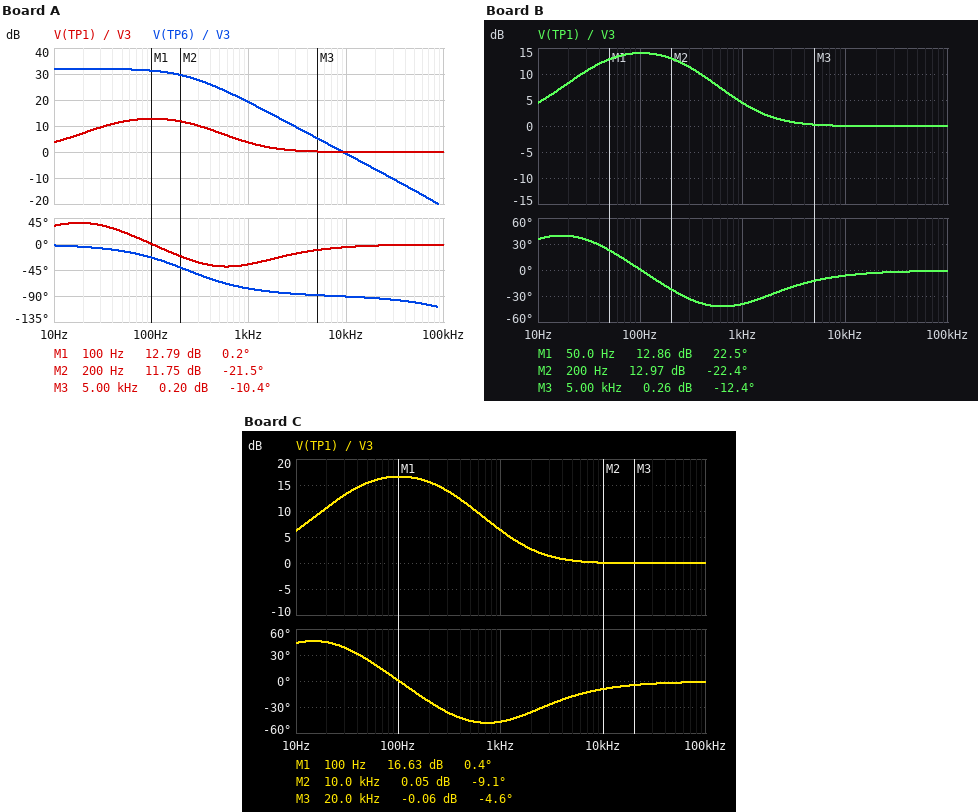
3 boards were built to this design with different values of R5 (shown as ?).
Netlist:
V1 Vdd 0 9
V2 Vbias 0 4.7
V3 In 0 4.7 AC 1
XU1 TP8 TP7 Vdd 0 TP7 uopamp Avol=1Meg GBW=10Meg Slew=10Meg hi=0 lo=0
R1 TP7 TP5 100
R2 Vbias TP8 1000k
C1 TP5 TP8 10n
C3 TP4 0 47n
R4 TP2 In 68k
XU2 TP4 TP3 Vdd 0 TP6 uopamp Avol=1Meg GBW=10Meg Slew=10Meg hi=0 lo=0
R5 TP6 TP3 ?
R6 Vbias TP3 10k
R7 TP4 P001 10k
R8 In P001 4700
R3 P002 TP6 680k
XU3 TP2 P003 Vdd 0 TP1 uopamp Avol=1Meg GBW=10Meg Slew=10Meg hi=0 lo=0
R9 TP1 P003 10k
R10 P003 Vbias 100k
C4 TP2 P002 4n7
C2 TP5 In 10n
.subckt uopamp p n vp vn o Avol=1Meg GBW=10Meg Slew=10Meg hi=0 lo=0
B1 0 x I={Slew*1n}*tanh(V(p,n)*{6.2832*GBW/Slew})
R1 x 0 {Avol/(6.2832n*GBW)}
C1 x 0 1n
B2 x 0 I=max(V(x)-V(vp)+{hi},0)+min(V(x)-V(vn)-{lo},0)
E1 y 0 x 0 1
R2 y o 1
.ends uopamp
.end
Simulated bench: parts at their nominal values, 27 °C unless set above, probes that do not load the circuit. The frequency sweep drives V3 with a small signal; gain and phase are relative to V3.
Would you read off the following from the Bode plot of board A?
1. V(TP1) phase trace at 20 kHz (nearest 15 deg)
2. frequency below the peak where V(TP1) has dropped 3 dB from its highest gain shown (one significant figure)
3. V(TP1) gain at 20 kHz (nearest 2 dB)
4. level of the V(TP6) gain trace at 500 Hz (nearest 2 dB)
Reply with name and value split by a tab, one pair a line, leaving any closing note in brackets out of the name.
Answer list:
V(TP1) phase trace at 20 kHz	0 deg
frequency below the peak where V(TP1) has dropped 3 dB from its highest gain shown	30 Hz
V(TP1) gain at 20 kHz	0 dB
level of the V(TP6) gain trace at 500 Hz	24 dB
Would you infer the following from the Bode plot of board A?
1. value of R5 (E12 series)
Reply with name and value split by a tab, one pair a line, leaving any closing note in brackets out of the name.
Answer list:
value of R5	390 kΩ
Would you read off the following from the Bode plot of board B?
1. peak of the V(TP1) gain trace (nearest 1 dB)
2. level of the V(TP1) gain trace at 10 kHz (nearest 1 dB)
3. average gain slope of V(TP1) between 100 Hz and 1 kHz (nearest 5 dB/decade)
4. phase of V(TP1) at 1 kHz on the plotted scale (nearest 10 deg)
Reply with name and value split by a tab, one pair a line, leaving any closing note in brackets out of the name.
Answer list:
peak of the V(TP1) gain trace	14 dB
level of the V(TP1) gain trace at 10 kHz	0 dB
average gain slope of V(TP1) between 100 Hz and 1 kHz	-10 dB/decade
phase of V(TP1) at 1 kHz on the plotted scale	-40 deg
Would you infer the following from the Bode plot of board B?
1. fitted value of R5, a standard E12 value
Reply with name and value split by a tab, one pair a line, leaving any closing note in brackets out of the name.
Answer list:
fitted value of R5, a standard E12 value	470 kΩ
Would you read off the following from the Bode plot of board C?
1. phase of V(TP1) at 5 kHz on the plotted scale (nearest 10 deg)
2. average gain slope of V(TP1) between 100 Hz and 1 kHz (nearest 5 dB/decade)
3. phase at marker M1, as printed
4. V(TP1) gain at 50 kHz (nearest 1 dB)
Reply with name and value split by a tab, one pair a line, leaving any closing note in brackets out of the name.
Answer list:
phase of V(TP1) at 5 kHz on the plotted scale	-20 deg
average gain slope of V(TP1) between 100 Hz and 1 kHz	-10 dB/decade
phase at marker M1, as printed	0.4 deg
V(TP1) gain at 50 kHz	0 dB
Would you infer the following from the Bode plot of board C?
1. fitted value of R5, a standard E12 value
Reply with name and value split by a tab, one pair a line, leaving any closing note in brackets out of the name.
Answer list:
fitted value of R5, a standard E12 value	680 kΩ
